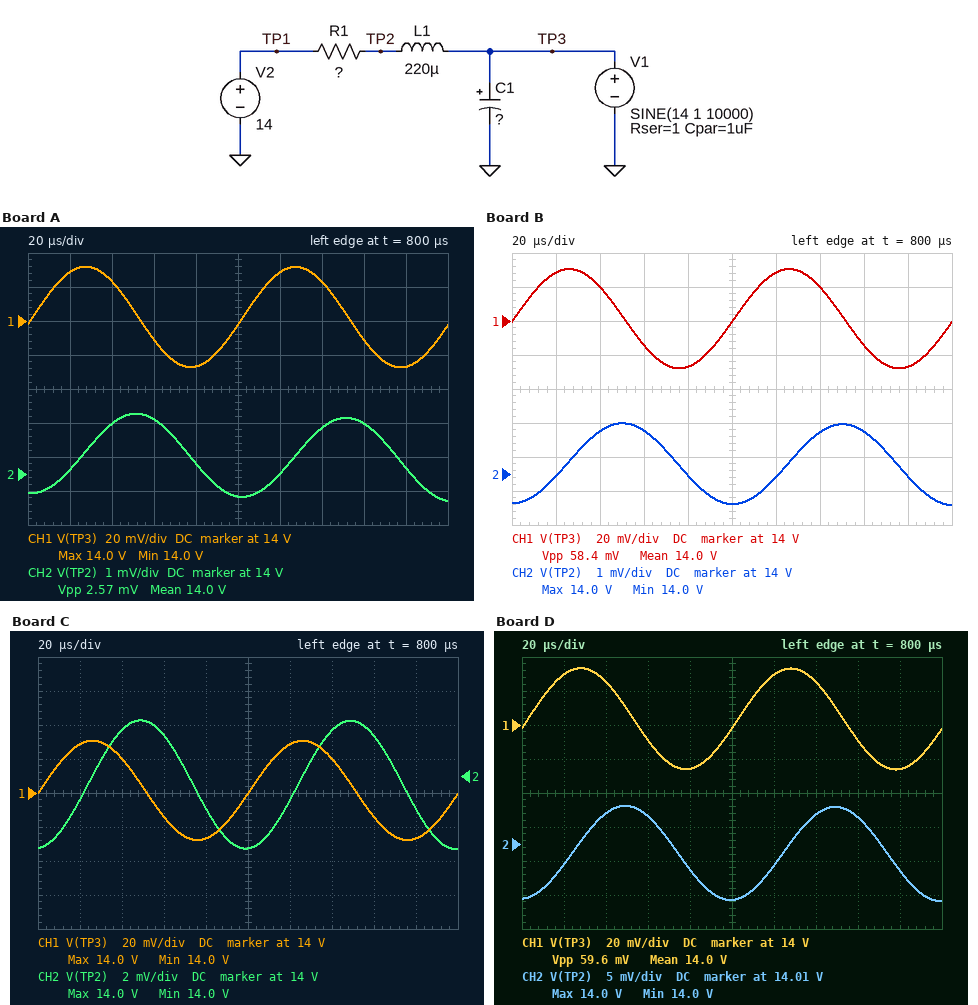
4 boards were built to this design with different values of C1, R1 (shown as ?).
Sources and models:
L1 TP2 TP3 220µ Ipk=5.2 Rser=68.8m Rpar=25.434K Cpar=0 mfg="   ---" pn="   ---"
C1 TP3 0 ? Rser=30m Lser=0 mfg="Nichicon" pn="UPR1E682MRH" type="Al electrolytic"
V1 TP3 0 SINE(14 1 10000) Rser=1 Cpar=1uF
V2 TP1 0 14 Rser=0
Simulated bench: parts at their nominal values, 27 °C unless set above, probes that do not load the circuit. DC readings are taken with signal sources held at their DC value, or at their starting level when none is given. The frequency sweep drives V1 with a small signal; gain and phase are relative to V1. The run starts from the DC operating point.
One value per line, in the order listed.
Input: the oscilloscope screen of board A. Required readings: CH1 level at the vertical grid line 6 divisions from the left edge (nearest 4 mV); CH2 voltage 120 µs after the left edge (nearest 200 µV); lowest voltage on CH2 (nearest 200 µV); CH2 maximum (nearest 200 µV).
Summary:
14.028 V
14.0020 V
14.0012 V
14.0038 V
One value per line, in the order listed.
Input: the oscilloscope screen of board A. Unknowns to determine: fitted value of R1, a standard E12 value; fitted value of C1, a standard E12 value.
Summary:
0.56 Ω
3.3 mF
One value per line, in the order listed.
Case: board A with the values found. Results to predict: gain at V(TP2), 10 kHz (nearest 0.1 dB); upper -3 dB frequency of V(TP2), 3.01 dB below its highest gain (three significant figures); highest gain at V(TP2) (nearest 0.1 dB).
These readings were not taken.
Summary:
-58.5 dB
131 Hz
-9.3 dB
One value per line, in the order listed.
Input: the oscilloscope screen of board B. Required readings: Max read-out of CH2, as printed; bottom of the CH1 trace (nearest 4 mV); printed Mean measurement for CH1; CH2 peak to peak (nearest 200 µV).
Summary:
14.0 V
13.972 V
14.0 V
2.4 mV
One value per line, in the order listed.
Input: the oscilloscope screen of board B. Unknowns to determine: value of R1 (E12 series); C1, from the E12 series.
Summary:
0.56 Ω
8.2 mF
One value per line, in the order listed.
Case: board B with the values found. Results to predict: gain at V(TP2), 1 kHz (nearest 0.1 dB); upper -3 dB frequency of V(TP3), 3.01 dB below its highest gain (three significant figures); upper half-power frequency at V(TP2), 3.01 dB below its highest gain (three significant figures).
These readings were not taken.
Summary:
-37.8 dB
50.2 Hz
49.6 Hz
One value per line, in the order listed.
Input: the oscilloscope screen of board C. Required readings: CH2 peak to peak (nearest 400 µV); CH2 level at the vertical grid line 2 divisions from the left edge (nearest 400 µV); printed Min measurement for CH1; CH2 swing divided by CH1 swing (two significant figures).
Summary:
7.6 mV
14.0048 V
14.0 V
0.13
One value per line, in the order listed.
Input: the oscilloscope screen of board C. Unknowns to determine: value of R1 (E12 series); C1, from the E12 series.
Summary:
1.8 Ω
8.2 mF
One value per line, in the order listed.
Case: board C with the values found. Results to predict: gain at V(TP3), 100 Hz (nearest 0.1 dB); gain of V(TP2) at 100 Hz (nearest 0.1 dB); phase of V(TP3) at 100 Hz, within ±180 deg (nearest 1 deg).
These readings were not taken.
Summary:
-14.8 dB
-15.2 dB
-65 deg
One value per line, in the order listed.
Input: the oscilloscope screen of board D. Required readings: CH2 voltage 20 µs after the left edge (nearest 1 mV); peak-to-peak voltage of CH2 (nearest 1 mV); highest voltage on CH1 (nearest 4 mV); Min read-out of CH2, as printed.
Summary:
14.002 V
14 mV
14.032 V
14.0 V
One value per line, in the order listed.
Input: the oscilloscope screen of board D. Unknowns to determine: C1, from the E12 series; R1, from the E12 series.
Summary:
2.7 mF
3.3 Ω
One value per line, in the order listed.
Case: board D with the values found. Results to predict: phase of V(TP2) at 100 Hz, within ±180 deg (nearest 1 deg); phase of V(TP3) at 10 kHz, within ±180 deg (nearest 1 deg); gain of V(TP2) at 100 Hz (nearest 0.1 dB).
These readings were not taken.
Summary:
-53 deg
-11 deg
-6.9 dB
